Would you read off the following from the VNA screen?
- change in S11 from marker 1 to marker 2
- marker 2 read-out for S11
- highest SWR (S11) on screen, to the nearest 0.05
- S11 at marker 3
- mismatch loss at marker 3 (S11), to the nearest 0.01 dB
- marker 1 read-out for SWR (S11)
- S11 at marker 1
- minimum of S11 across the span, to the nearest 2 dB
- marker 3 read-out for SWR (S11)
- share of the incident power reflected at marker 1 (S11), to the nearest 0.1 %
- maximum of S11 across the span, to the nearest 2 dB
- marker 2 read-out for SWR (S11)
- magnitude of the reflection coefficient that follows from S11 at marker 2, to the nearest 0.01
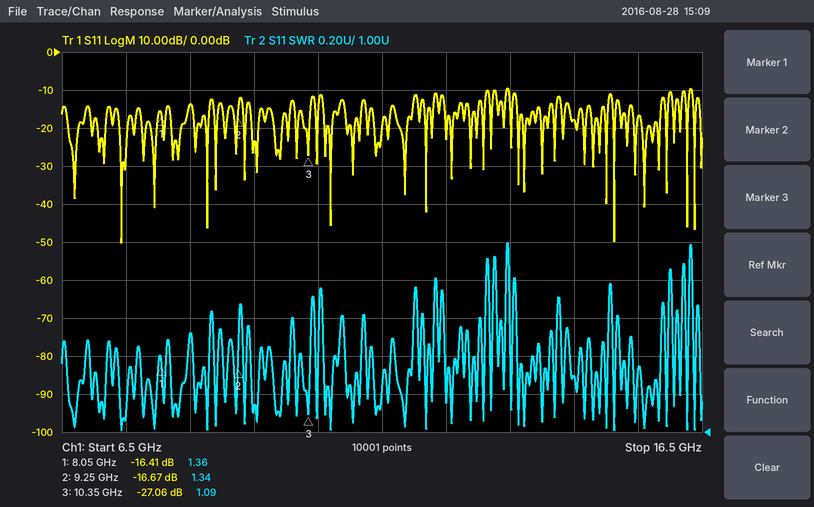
-0.26 dB
-16.67 dB
2.00
-27.06 dB
0.01 dB
1.36
-16.41 dB
-50 dB
1.09
2.3 %
-10 dB
1.34
0.15
